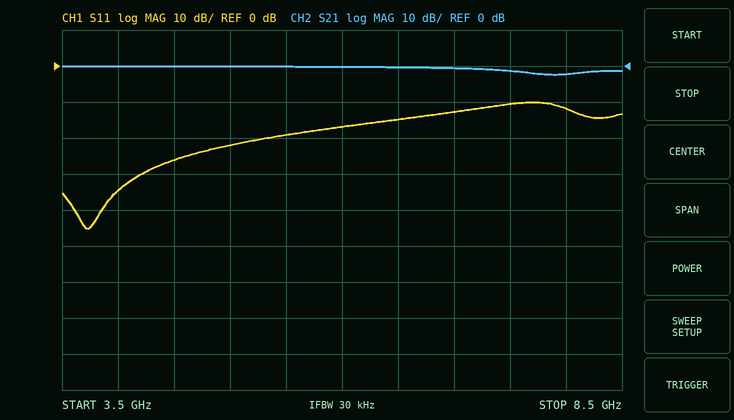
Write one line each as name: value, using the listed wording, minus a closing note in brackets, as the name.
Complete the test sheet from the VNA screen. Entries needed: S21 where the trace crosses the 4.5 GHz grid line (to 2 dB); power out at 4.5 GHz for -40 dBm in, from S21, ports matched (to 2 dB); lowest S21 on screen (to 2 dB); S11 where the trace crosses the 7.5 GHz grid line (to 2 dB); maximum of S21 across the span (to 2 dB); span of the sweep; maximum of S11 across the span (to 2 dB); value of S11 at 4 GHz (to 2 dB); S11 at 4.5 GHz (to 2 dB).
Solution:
S21 where the trace crosses the 4.5 GHz grid line: 0 dB
power out at 4.5 GHz for -40 dBm in, from S21, ports matched: -40 dBm
lowest S21 on screen: -2 dB
S11 where the trace crosses the 7.5 GHz grid line: -10 dB
maximum of S21 across the span: 0 dB
span of the sweep: 5 GHz
maximum of S11 across the span: -10 dB
value of S11 at 4 GHz: -34 dB
S11 at 4.5 GHz: -26 dB
